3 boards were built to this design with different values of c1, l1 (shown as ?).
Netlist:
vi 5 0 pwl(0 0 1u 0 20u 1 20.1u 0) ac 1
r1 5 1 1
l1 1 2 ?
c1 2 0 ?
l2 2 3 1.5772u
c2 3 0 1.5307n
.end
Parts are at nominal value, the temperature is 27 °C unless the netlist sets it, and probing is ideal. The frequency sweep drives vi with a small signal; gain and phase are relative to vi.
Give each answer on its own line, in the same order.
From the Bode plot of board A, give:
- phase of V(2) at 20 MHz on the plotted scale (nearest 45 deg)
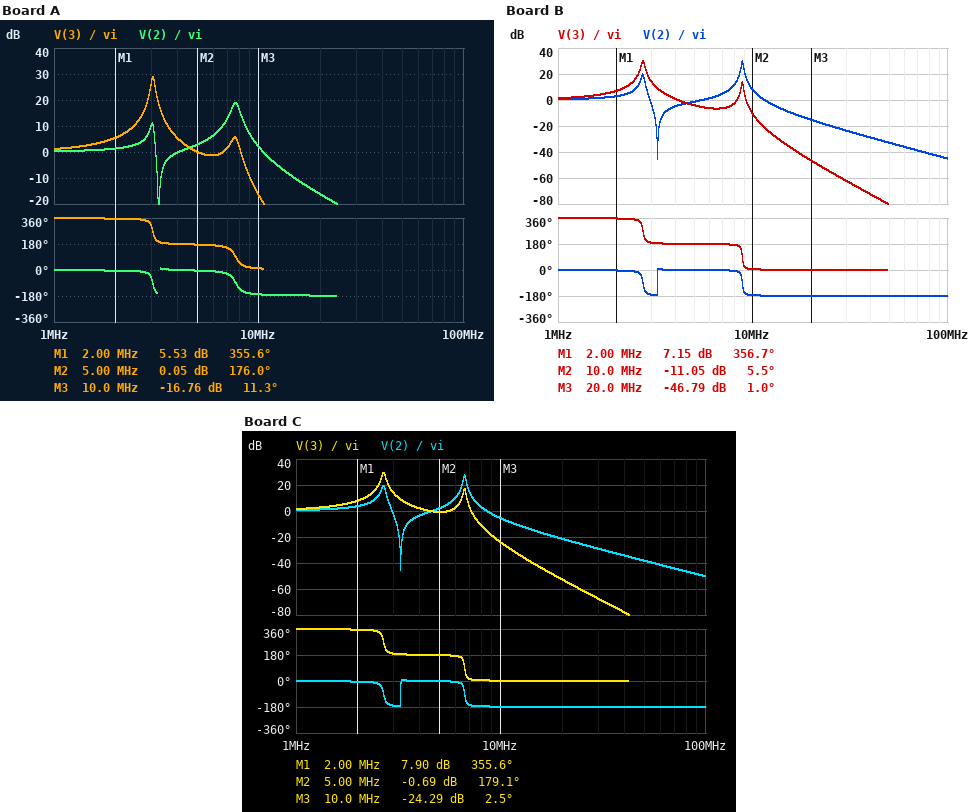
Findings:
-180 deg
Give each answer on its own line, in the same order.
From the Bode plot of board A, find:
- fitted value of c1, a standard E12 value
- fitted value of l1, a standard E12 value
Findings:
2.7 nF
180 nH
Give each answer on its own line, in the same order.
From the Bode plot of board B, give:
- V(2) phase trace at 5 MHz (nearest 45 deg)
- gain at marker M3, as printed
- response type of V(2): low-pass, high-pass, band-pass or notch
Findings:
0 deg
-46.79 dB
band-pass
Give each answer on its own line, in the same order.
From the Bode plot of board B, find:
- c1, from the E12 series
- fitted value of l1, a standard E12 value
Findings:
820 pF
560 nH
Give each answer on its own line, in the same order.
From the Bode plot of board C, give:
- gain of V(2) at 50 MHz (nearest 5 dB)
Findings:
-40 dB
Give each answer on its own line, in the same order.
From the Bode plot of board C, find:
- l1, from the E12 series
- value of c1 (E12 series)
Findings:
560 nH
1.5 nF
